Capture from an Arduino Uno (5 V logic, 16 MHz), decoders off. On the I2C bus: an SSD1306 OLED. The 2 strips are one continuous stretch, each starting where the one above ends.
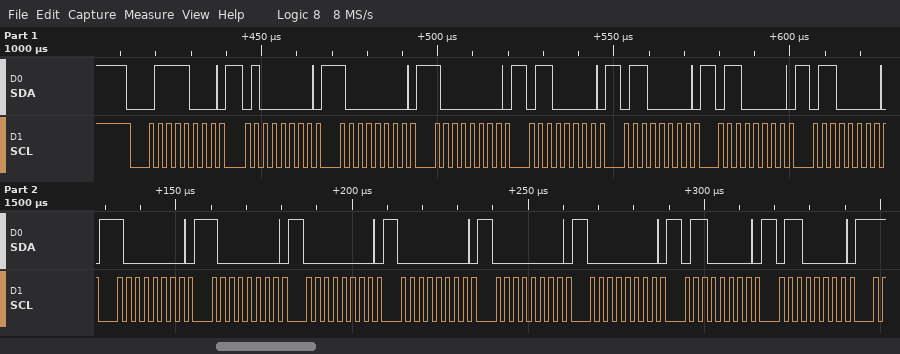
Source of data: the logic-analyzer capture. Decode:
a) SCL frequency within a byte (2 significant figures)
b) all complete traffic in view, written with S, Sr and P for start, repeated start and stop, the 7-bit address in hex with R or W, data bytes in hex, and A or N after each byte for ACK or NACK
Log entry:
400 kHz
S 3CW A 40 A 80 A 80 A 60 A 60 A 60 A 60 A 80 A 80 A 00 A 00 A 00 A 00 A 60 A 60 A
